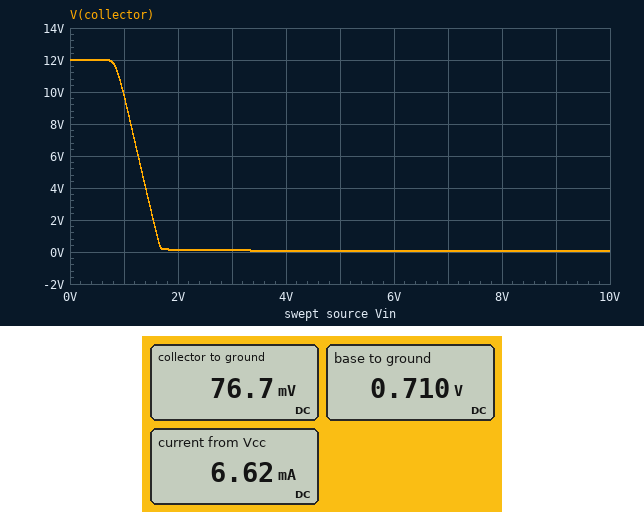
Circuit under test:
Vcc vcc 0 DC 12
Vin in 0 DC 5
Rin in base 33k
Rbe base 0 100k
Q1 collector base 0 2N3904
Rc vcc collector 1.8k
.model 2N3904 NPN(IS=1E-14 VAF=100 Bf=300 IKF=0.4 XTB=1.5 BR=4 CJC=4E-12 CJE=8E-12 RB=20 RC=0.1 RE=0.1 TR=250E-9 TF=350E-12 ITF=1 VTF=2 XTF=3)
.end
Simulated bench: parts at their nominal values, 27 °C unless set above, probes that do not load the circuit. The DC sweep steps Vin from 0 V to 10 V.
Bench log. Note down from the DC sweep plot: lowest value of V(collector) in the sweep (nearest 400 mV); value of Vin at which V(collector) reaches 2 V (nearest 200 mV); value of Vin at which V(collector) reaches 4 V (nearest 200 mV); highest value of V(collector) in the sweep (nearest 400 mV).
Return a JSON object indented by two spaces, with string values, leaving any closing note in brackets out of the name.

{
  "lowest value of V(collector) in the sweep": "0 V",
  "value of Vin at which V(collector) reaches 2 V": "1.6 V",
  "value of Vin at which V(collector) reaches 4 V": "1.4 V",
  "highest value of V(collector) in the sweep": "12.0 V"
}
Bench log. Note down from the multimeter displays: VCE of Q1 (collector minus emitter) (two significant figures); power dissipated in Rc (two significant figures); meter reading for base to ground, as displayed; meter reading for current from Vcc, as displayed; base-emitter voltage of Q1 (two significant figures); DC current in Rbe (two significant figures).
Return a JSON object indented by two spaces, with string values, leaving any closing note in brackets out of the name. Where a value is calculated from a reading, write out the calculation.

{
  "VCE of Q1 (collector minus emitter)": "76.7 mV = 77 mV",
  "power dissipated in Rc": "(12 V - 76.7 mV)^2 / 1.8 kΩ = 79 mW",
  "meter reading for base to ground, as displayed": "0.710 V",
  "meter reading for current from Vcc, as displayed": "6.62 mA",
  "base-emitter voltage of Q1": "710 mV = 710 mV",
  "DC current in Rbe": "(710 mV) / 100 kΩ = 7.1 µA"
}
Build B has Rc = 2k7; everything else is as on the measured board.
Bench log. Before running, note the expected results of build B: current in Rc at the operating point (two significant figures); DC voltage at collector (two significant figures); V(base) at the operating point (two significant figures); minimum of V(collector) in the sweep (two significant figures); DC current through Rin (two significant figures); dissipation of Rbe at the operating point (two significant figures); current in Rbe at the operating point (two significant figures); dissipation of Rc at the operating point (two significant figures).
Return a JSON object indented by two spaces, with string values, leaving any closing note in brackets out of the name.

{
  "current in Rc at the operating point": "4.4 mA",
  "DC voltage at collector": "65 mV",
  "V(base) at the operating point": "700 mV",
  "minimum of V(collector) in the sweep": "46 mV",
  "DC current through Rin": "130 µA",
  "dissipation of Rbe at the operating point": "4.9 µW",
  "current in Rbe at the operating point": "7.0 µA",
  "dissipation of Rc at the operating point": "53 mW"
}
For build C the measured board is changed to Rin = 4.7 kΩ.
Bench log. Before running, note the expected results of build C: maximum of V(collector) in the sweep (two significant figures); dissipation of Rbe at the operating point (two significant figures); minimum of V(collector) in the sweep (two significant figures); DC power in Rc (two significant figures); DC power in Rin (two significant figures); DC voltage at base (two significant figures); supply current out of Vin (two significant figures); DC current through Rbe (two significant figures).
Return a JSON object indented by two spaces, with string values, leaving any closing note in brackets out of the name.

{
  "maximum of V(collector) in the sweep": "12 V",
  "dissipation of Rbe at the operating point": "5.4 µW",
  "minimum of V(collector) in the sweep": "22 mV",
  "DC power in Rc": "80 mW",
  "DC power in Rin": "3.9 mW",
  "DC voltage at base": "740 mV",
  "supply current out of Vin": "910 µA",
  "DC current through Rbe": "7.4 µA"
}
